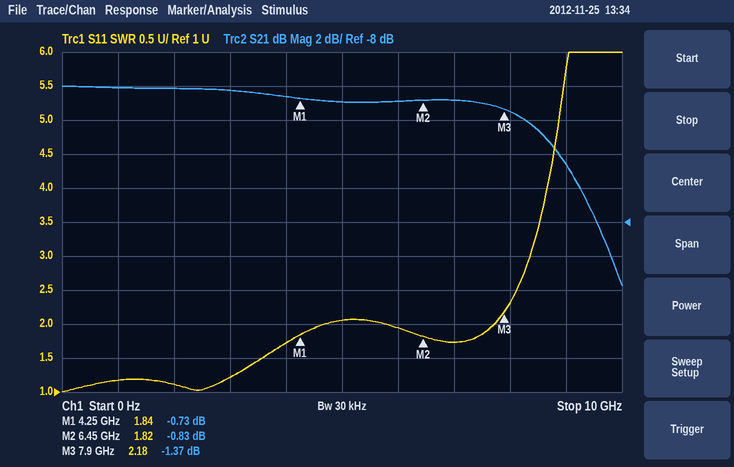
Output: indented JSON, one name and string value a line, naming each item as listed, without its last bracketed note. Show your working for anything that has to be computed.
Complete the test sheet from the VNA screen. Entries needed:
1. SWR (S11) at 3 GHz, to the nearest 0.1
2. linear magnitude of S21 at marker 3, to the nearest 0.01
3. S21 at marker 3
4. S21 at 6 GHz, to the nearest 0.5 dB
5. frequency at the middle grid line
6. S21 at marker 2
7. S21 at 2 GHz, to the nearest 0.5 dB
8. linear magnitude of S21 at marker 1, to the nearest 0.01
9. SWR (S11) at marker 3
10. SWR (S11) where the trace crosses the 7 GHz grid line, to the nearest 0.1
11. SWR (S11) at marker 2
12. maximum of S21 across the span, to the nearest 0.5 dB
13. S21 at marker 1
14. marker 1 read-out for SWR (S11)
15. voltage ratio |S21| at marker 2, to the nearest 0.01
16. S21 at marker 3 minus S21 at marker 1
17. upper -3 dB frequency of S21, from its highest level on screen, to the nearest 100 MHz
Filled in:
{
  "SWR (S11) at 3 GHz, to the nearest 0.1": "1.2",
  "linear magnitude of S21 at marker 3, to the nearest 0.01": "10^(-1.37/20) ≈ 0.85",
  "S21 at marker 3": "-1.37 dB",
  "S21 at 6 GHz, to the nearest 0.5 dB": "-1.0 dB",
  "frequency at the middle grid line": "5 GHz",
  "S21 at marker 2": "-0.83 dB",
  "S21 at 2 GHz, to the nearest 0.5 dB": "0.0 dB",
  "linear magnitude of S21 at marker 1, to the nearest 0.01": "10^(-0.73/20) ≈ 0.92",
  "SWR (S11) at marker 3": "2.18",
  "SWR (S11) where the trace crosses the 7 GHz grid line, to the nearest 0.1": "1.7",
  "SWR (S11) at marker 2": "1.82",
  "maximum of S21 across the span, to the nearest 0.5 dB": "0.0 dB",
  "S21 at marker 1": "-0.73 dB",
  "marker 1 read-out for SWR": "1.84",
  "voltage ratio |S21| at marker 2, to the nearest 0.01": "10^(-0.83/20) ≈ 0.91",
  "S21 at marker 3 minus S21 at marker 1": "-1.37 − (-0.73) = -0.64 dB",
  "upper -3 dB frequency of S21, from its highest level on screen, to the nearest 100 MHz": "8.6 GHz"
}
